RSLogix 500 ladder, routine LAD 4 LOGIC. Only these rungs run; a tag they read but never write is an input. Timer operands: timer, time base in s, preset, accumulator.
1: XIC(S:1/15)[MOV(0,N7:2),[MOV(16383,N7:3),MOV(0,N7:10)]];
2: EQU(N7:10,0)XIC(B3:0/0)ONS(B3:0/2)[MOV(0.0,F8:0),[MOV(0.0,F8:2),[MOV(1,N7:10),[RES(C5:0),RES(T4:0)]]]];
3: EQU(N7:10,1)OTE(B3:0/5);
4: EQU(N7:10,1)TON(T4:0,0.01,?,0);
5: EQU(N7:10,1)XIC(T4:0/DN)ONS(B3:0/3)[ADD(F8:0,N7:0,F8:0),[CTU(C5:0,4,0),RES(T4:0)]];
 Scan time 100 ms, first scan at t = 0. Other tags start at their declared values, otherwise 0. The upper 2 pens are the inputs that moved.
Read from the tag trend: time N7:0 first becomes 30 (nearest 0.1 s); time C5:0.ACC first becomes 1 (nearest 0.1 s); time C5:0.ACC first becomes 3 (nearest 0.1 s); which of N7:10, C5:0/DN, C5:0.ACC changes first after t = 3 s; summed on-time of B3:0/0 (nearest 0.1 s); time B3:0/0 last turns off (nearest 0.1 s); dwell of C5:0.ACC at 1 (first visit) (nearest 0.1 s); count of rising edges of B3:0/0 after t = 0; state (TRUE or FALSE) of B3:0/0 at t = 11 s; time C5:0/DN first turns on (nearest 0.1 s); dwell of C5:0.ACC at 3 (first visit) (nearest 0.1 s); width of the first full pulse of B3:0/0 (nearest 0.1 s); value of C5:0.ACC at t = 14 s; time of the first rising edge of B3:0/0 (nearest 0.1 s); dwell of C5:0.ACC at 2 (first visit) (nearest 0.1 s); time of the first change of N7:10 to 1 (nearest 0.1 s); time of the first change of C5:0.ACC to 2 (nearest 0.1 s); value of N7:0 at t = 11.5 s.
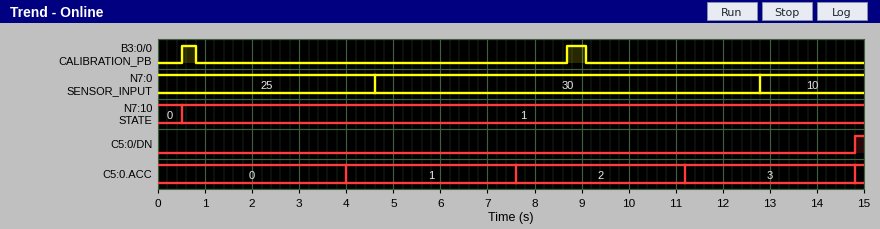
4.6 s
4.0 s
11.2 s
C5:0.ACC
0.7 s
9.1 s
3.6 s
2
FALSE
14.8 s
3.6 s
0.3 s
3
0.5 s
3.6 s
0.5 s
7.6 s
30
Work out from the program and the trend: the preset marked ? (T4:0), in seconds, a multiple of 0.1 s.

3.5 s
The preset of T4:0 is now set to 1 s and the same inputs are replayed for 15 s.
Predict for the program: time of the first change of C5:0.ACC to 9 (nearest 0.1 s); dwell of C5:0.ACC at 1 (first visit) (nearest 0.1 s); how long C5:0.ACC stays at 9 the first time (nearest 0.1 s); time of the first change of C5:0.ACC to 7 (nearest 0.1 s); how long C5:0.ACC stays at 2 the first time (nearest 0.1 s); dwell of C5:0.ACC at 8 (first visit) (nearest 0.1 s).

10.3 s
1.1 s
1.1 s
8.1 s
1.1 s
1.1 s
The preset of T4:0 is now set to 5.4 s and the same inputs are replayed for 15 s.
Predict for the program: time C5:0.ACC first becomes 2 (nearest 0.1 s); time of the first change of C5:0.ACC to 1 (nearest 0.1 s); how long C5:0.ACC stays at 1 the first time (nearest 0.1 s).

11.4 s
5.9 s
5.5 s
